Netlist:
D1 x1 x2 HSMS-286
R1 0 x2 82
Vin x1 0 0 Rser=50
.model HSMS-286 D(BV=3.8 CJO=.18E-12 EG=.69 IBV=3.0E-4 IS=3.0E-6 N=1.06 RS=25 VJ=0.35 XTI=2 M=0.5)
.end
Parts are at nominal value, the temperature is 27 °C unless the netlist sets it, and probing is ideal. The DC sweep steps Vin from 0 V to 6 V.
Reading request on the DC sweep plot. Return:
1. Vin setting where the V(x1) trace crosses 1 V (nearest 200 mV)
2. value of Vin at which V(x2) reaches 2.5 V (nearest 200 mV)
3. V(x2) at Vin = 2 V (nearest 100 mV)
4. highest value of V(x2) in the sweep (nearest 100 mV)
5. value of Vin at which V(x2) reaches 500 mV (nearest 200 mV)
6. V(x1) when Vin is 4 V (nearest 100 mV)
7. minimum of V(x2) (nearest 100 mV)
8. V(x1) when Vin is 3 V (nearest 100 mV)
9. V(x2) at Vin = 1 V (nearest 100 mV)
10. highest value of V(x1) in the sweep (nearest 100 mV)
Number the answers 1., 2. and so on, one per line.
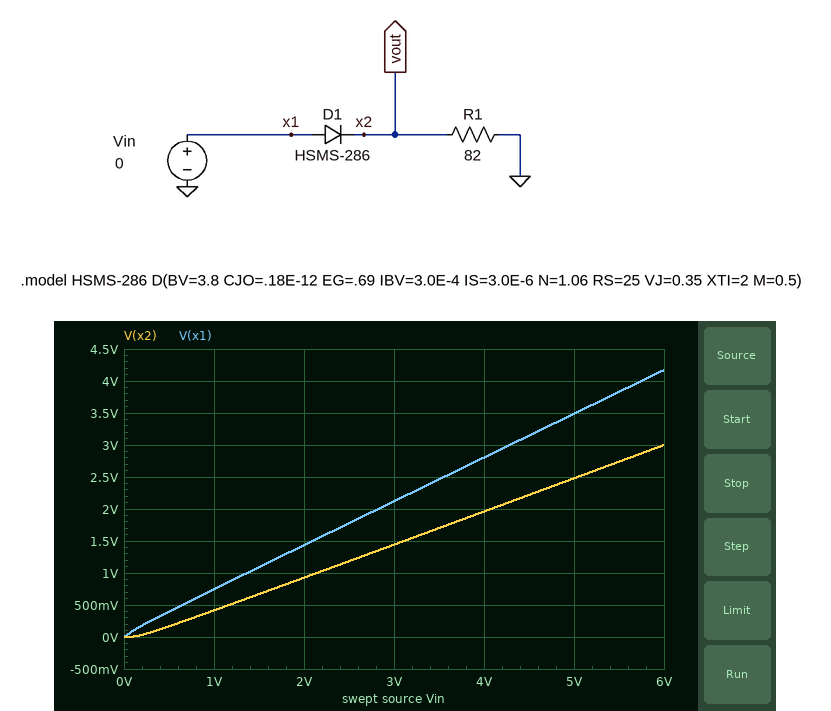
1. 1.4 V
2. 5.0 V
3. 900 mV
4. 3.0 V
5. 1.2 V
6. 2.8 V
7. 0 V
8. 2.1 V
9. 400 mV
10. 4.2 V
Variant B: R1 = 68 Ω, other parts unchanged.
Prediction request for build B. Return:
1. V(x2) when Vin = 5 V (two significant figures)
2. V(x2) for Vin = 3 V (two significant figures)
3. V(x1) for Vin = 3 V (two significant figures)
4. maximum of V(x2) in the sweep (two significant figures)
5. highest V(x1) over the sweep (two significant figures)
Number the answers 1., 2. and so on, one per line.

1. 2.3 V
2. 1.3 V
3. 2.0 V
4. 2.7 V
5. 4.0 V
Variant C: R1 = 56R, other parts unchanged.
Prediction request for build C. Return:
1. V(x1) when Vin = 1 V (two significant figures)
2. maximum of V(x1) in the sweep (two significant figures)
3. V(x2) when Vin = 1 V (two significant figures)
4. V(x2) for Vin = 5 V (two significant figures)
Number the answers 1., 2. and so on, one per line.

1. 700 mV
2. 3.8 V
3. 340 mV
4. 2.0 V
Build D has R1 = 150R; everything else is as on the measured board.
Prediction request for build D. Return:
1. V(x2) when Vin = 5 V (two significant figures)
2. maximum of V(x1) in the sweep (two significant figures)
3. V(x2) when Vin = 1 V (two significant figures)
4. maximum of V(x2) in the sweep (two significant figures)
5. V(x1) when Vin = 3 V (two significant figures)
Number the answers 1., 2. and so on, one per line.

1. 3.2 V
2. 4.7 V
3. 540 mV
4. 3.8 V
5. 2.4 V
